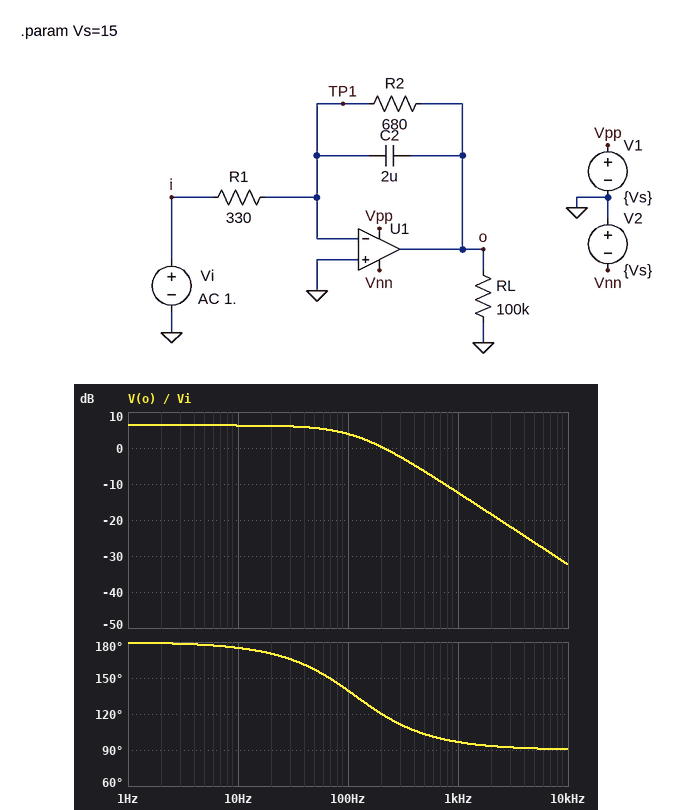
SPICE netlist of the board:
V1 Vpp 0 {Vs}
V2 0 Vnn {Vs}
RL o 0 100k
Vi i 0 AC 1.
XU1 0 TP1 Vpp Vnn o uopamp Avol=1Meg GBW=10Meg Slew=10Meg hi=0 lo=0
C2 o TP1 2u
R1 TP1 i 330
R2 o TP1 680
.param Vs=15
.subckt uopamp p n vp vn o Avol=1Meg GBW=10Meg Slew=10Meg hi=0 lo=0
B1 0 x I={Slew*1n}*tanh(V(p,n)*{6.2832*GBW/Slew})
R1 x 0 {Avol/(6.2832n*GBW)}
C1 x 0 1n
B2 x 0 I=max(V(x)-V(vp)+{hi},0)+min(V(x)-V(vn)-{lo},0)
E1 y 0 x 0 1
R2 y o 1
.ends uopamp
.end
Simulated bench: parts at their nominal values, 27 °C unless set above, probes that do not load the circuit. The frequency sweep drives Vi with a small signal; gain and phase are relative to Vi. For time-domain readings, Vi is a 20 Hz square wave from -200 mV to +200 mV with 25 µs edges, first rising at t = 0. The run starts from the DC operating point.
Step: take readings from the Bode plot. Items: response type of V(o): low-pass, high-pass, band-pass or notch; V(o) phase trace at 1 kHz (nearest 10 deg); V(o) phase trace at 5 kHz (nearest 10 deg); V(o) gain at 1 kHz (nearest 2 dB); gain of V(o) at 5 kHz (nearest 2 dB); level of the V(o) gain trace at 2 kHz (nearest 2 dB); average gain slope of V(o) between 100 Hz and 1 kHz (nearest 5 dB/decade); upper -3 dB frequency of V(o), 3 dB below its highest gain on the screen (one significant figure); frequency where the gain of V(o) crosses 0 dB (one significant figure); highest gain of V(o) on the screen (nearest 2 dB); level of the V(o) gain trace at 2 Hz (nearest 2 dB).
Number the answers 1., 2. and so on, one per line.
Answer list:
1. low-pass
2. 100 deg
3. 90 deg
4. -12 dB
5. -26 dB
6. -18 dB
7. -15 dB/decade
8. 100 Hz
9. 200 Hz
10. 6 dB
11. 6 dB
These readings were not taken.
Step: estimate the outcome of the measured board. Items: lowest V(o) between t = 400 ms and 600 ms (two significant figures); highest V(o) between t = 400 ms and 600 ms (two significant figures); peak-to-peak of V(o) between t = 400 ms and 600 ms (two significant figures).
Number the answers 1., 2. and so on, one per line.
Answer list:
1. -410 mV
2. 410 mV
3. 820 mV
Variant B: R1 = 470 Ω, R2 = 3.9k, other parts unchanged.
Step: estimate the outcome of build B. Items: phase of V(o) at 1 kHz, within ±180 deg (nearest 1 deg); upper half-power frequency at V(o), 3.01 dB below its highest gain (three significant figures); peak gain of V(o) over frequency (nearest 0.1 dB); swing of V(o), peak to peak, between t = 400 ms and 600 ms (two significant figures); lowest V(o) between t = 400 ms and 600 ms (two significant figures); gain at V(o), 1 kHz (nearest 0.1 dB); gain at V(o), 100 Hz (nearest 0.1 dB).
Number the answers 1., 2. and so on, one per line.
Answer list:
1. 91 deg
2. 20.4 Hz
3. 18.4 dB
4. 3.1 V
5. -1.5 V
6. -15.4 dB
7. 4.4 dB
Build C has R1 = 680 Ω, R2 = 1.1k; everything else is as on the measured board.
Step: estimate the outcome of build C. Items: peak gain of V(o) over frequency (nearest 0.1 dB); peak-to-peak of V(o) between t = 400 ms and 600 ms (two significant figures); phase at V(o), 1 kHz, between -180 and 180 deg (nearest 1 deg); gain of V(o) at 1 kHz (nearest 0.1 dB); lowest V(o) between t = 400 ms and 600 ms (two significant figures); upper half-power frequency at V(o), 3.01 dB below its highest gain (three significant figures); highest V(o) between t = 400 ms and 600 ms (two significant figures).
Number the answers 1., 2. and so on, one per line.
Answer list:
1. 4.2 dB
2. 650 mV
3. 94 deg
4. -18.7 dB
5. -320 mV
6. 72.3 Hz
7. 320 mV
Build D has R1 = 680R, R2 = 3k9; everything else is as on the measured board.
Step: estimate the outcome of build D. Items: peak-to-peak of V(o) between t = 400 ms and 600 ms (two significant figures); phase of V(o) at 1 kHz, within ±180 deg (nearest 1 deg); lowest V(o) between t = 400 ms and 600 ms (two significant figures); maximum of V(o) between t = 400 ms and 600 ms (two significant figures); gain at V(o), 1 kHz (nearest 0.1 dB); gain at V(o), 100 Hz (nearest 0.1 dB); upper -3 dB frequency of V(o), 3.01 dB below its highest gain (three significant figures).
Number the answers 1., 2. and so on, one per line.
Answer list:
1. 2.1 V
2. 91 deg
3. -1.1 V
4. 1.1 V
5. -18.6 dB
6. 1.2 dB
7. 20.4 Hz
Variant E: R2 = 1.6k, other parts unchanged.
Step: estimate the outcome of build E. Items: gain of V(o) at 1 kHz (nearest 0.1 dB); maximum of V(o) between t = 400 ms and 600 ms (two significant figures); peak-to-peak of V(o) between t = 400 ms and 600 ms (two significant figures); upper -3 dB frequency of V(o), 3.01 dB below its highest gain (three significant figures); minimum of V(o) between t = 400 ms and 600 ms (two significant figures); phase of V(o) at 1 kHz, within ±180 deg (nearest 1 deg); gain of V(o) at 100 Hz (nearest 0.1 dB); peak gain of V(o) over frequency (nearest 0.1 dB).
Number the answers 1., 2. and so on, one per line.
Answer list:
1. -12.4 dB
2. 970 mV
3. 1.9 V
4. 49.7 Hz
5. -970 mV
6. 93 deg
7. 6.7 dB
8. 13.7 dB
